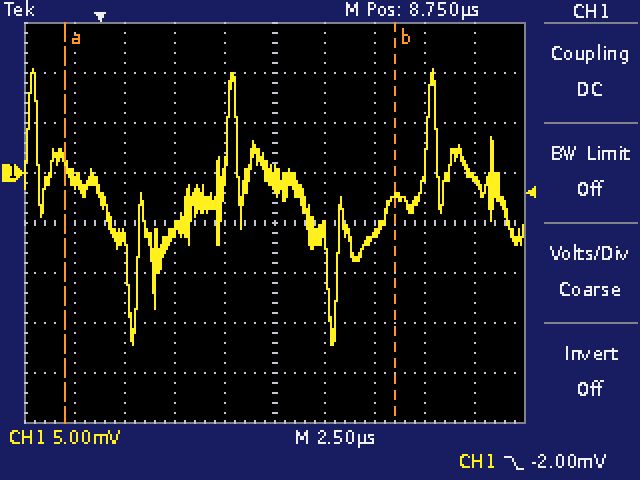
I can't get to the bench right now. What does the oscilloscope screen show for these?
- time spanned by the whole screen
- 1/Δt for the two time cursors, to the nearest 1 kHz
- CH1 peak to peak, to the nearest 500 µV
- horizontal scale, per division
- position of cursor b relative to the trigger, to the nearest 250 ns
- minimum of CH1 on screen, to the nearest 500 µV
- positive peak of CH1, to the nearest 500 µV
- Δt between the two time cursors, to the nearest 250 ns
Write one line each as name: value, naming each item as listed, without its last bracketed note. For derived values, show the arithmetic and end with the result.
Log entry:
time spanned by the whole screen: 25 µs
1/Δt for the two time cursors, to the nearest 1 kHz: 1 / 16.50 µs ≈ 61 kHz
CH1 peak to peak, to the nearest 500 µV: 10.5 mV − (-17.0 mV) = 27.5 mV
horizontal scale, per division: 2.5 µs
position of cursor b relative to the trigger, to the nearest 250 ns: +14.75 µs
minimum of CH1 on screen, to the nearest 500 µV: -17.0 mV
positive peak of CH1, to the nearest 500 µV: 10.5 mV
Δt between the two time cursors, to the nearest 250 ns: 16.50 µs
